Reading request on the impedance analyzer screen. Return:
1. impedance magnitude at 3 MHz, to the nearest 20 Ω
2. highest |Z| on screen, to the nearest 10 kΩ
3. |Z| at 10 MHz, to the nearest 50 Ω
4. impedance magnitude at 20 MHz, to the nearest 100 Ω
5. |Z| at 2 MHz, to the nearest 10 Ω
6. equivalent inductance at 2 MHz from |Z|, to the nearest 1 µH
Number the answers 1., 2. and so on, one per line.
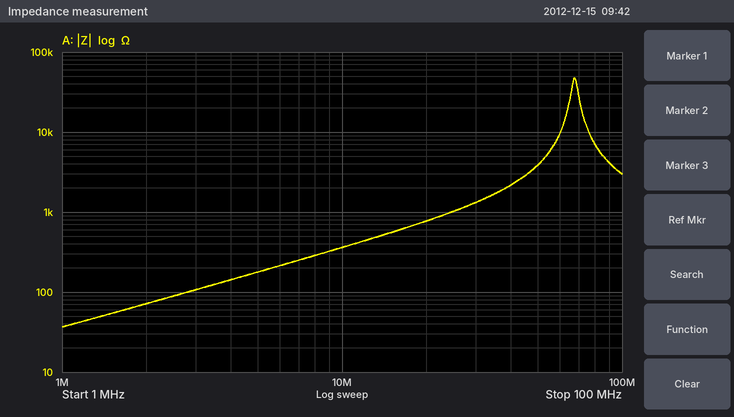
1. 100 Ω
2. 50 kΩ
3. 350 Ω
4. 800 Ω
5. 70 Ω
6. 6 µH
